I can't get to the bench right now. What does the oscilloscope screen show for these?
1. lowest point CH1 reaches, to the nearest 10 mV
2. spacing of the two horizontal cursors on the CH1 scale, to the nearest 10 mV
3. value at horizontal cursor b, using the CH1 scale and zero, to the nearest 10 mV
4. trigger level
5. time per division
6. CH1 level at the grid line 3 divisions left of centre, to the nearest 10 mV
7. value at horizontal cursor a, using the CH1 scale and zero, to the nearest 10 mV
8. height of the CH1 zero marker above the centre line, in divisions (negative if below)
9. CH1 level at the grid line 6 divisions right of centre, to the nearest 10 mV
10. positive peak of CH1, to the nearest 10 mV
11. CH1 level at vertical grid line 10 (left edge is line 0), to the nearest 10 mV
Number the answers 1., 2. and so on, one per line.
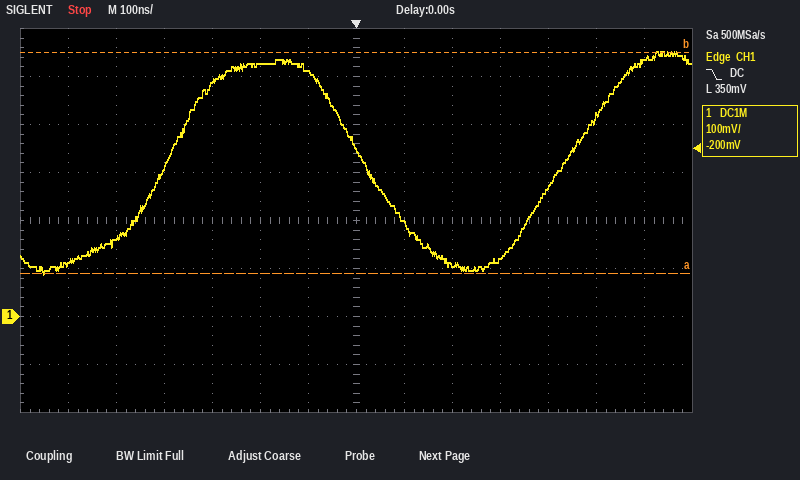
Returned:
1. 90 mV
2. 460 mV
3. 550 mV
4. 350 mV
5. 100 ns
6. 490 mV
7. 90 mV
8. -2.0 div
9. 530 mV
10. 550 mV
11. 120 mV
